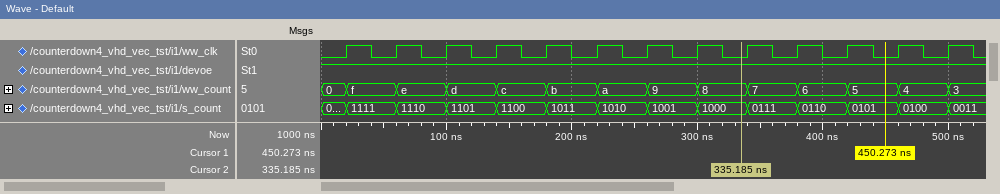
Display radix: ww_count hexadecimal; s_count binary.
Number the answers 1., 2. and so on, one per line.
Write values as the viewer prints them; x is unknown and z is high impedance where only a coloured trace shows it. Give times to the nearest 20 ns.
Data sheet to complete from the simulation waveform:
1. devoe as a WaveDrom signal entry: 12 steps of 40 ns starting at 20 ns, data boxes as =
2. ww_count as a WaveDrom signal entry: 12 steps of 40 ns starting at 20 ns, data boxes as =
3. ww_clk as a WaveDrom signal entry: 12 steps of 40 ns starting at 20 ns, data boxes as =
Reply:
1. {name: 'devoe', wave: '1...........'}
2. {name: 'ww_count', wave: '============', data: 'f e d c b a 9 8 7 6 5 4'}
3. {name: 'ww_clk', wave: 'p...........'}
